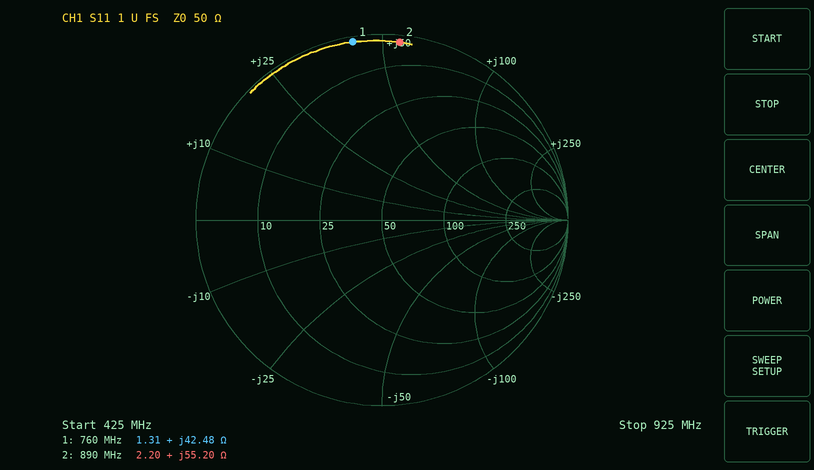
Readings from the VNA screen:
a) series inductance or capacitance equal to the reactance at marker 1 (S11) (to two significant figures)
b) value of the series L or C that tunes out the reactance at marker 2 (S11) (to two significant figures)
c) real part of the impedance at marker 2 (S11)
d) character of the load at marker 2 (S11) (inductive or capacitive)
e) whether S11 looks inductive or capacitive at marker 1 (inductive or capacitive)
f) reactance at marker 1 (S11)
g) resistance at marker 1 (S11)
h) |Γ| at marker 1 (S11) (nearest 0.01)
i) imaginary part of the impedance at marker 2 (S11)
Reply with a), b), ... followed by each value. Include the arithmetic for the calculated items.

a) L = 42.48 Ω/(2π × 760 MHz) ≈ 8.9 nH
b) C = 1/(2π × 890 MHz × 55.2 Ω) ≈ 3.2 pF
c) 2.20 Ω
d) inductive
e) inductive
f) +42.48 Ω
g) 1.31 Ω
h) 0.97
i) +55.20 Ω
